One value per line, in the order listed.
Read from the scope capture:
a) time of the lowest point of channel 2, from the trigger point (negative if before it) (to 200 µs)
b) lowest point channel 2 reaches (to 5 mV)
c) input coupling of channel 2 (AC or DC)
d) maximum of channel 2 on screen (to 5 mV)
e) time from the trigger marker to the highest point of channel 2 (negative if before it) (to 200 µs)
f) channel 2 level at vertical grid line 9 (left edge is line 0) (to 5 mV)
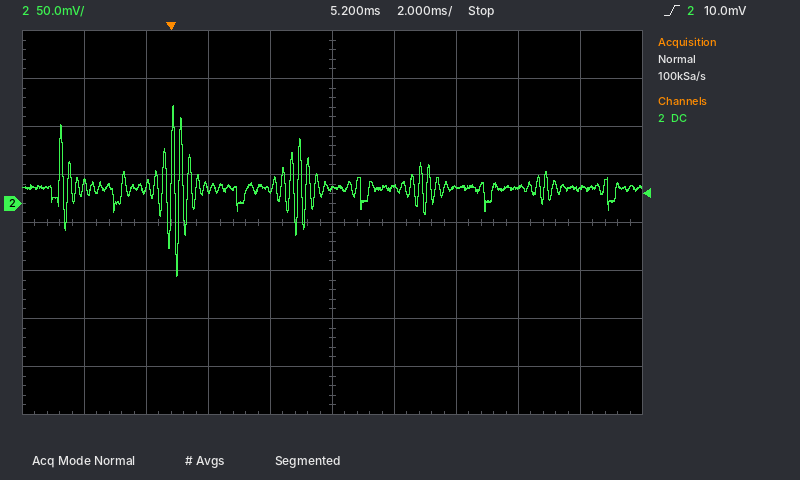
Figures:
+200 µs
-75 mV
DC
100 mV
0.0 ms
15 mV
